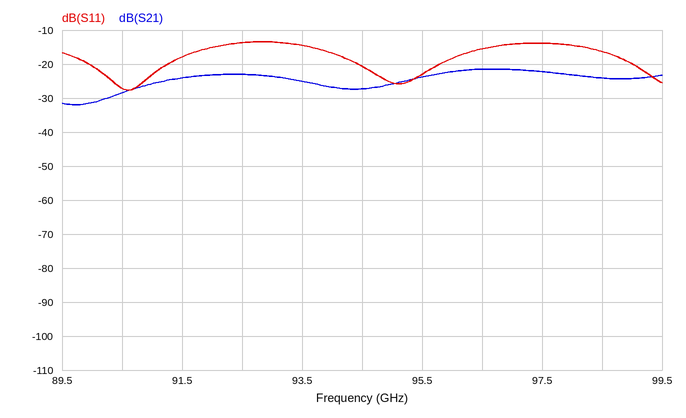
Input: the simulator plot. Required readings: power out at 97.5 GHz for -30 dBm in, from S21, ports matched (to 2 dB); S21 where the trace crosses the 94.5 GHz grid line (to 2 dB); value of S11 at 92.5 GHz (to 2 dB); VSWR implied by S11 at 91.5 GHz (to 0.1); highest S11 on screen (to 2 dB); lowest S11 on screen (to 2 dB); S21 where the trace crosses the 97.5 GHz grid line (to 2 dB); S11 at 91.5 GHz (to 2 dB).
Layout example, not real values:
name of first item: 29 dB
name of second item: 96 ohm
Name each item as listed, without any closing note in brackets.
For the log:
power out at 97.5 GHz for -30 dBm in, from S21, ports matched: -52 dBm
S21 where the trace crosses the 94.5 GHz grid line: -28 dB
value of S11 at 92.5 GHz: -14 dB
VSWR implied by S11 at 91.5 GHz: 1.3
highest S11 on screen: -14 dB
lowest S11 on screen: -28 dB
S21 where the trace crosses the 97.5 GHz grid line: -22 dB
S11 at 91.5 GHz: -18 dB
